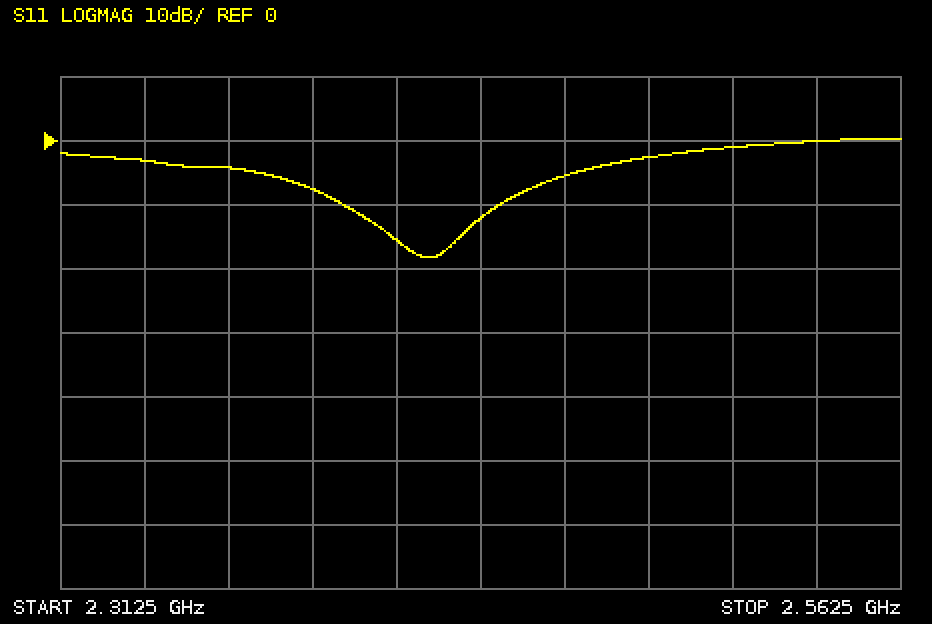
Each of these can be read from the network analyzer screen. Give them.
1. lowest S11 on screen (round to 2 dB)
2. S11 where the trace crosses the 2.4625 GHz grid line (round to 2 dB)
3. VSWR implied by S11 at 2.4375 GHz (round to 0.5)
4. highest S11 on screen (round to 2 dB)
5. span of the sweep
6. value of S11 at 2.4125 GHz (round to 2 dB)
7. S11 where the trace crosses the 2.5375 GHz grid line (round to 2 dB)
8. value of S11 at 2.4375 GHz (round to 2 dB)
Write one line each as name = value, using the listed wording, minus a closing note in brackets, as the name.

lowest S11 on screen = -18 dB
S11 where the trace crosses the 2.4625 GHz grid line = -6 dB
VSWR implied by S11 at 2.4375 GHz = 1.5
highest S11 on screen = 0 dB
span of the sweep = 250 MHz
value of S11 at 2.4125 GHz = -16 dB
S11 where the trace crosses the 2.5375 GHz grid line = 0 dB
value of S11 at 2.4375 GHz = -12 dB
